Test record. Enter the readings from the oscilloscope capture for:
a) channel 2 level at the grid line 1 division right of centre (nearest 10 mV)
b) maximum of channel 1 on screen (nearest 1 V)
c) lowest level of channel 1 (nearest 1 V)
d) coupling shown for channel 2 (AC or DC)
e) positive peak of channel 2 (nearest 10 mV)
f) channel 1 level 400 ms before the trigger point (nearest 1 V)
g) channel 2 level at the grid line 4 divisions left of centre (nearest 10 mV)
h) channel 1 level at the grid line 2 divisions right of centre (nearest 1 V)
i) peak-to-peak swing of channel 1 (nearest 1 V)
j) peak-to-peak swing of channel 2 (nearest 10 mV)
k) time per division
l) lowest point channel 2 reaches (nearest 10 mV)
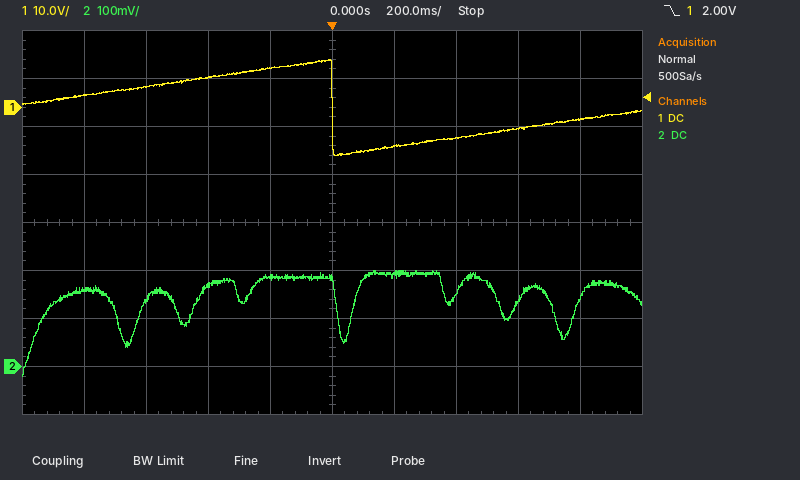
190 mV
10 V
-10 V
DC
200 mV
6 V
160 mV
-6 V
20 V
220 mV
200 ms
-20 mV
